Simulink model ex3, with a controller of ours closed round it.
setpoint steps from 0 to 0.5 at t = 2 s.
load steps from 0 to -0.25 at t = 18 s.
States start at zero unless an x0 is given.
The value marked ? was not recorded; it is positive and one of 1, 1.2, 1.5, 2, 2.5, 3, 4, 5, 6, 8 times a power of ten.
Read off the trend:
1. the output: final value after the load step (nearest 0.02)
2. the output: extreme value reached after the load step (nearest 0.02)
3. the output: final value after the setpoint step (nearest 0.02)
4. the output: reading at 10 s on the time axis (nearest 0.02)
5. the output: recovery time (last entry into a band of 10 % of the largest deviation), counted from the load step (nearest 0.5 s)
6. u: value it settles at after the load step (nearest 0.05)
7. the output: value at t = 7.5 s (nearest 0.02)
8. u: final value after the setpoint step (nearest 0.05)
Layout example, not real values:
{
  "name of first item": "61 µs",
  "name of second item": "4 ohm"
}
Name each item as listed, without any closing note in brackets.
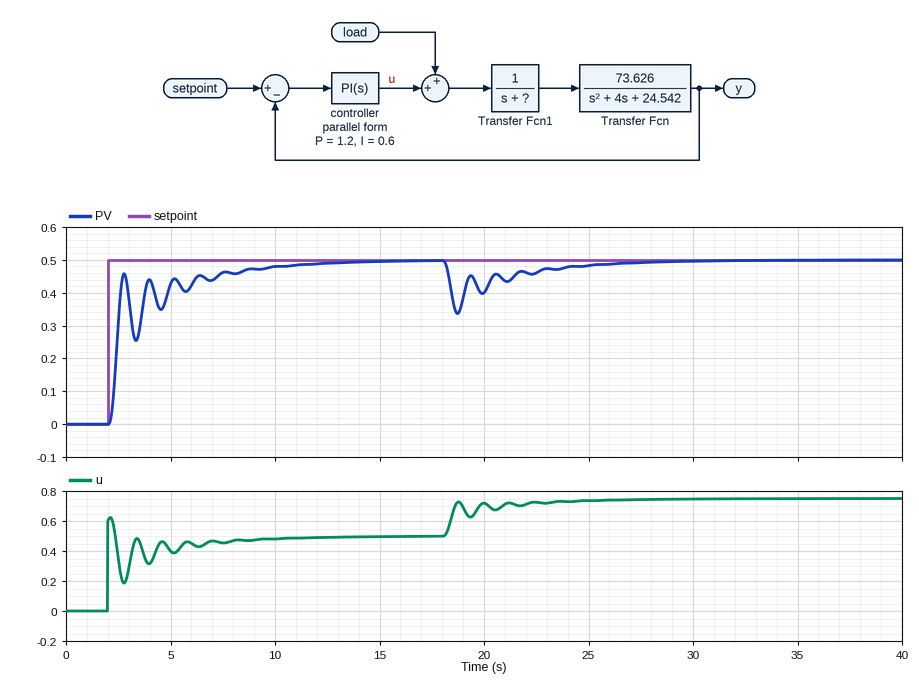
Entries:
{
  "the output: final value after the load step": "0.50",
  "the output: extreme value reached after the load step": "0.34",
  "the output: final value after the setpoint step": "0.50",
  "the output: reading at 10 s on the time axis": "0.48",
  "the output: recovery time (last entry into a band of 10 % of the largest deviation), counted from the load step": "7.0 s",
  "u: value it settles at after the load step": "0.75",
  "the output: value at t = 7.5 s": "0.46",
  "u: final value after the setpoint step": "0.50"
}
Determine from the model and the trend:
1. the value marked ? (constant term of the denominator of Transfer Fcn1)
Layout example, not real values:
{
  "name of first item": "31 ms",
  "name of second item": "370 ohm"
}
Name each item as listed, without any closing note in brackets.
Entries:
{
  "the value marked ?": "3"
}
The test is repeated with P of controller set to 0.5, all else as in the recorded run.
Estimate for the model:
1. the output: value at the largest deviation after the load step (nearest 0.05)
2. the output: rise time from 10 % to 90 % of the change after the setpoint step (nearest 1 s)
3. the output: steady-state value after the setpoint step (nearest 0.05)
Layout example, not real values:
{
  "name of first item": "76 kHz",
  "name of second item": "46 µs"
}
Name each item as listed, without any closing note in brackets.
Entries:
{
  "the output: value at the largest deviation after the load step": "0.30",
  "the output: rise time from 10 % to 90 % of the change after the setpoint step": "4 s",
  "the output: steady-state value after the setpoint step": "0.50"
}
